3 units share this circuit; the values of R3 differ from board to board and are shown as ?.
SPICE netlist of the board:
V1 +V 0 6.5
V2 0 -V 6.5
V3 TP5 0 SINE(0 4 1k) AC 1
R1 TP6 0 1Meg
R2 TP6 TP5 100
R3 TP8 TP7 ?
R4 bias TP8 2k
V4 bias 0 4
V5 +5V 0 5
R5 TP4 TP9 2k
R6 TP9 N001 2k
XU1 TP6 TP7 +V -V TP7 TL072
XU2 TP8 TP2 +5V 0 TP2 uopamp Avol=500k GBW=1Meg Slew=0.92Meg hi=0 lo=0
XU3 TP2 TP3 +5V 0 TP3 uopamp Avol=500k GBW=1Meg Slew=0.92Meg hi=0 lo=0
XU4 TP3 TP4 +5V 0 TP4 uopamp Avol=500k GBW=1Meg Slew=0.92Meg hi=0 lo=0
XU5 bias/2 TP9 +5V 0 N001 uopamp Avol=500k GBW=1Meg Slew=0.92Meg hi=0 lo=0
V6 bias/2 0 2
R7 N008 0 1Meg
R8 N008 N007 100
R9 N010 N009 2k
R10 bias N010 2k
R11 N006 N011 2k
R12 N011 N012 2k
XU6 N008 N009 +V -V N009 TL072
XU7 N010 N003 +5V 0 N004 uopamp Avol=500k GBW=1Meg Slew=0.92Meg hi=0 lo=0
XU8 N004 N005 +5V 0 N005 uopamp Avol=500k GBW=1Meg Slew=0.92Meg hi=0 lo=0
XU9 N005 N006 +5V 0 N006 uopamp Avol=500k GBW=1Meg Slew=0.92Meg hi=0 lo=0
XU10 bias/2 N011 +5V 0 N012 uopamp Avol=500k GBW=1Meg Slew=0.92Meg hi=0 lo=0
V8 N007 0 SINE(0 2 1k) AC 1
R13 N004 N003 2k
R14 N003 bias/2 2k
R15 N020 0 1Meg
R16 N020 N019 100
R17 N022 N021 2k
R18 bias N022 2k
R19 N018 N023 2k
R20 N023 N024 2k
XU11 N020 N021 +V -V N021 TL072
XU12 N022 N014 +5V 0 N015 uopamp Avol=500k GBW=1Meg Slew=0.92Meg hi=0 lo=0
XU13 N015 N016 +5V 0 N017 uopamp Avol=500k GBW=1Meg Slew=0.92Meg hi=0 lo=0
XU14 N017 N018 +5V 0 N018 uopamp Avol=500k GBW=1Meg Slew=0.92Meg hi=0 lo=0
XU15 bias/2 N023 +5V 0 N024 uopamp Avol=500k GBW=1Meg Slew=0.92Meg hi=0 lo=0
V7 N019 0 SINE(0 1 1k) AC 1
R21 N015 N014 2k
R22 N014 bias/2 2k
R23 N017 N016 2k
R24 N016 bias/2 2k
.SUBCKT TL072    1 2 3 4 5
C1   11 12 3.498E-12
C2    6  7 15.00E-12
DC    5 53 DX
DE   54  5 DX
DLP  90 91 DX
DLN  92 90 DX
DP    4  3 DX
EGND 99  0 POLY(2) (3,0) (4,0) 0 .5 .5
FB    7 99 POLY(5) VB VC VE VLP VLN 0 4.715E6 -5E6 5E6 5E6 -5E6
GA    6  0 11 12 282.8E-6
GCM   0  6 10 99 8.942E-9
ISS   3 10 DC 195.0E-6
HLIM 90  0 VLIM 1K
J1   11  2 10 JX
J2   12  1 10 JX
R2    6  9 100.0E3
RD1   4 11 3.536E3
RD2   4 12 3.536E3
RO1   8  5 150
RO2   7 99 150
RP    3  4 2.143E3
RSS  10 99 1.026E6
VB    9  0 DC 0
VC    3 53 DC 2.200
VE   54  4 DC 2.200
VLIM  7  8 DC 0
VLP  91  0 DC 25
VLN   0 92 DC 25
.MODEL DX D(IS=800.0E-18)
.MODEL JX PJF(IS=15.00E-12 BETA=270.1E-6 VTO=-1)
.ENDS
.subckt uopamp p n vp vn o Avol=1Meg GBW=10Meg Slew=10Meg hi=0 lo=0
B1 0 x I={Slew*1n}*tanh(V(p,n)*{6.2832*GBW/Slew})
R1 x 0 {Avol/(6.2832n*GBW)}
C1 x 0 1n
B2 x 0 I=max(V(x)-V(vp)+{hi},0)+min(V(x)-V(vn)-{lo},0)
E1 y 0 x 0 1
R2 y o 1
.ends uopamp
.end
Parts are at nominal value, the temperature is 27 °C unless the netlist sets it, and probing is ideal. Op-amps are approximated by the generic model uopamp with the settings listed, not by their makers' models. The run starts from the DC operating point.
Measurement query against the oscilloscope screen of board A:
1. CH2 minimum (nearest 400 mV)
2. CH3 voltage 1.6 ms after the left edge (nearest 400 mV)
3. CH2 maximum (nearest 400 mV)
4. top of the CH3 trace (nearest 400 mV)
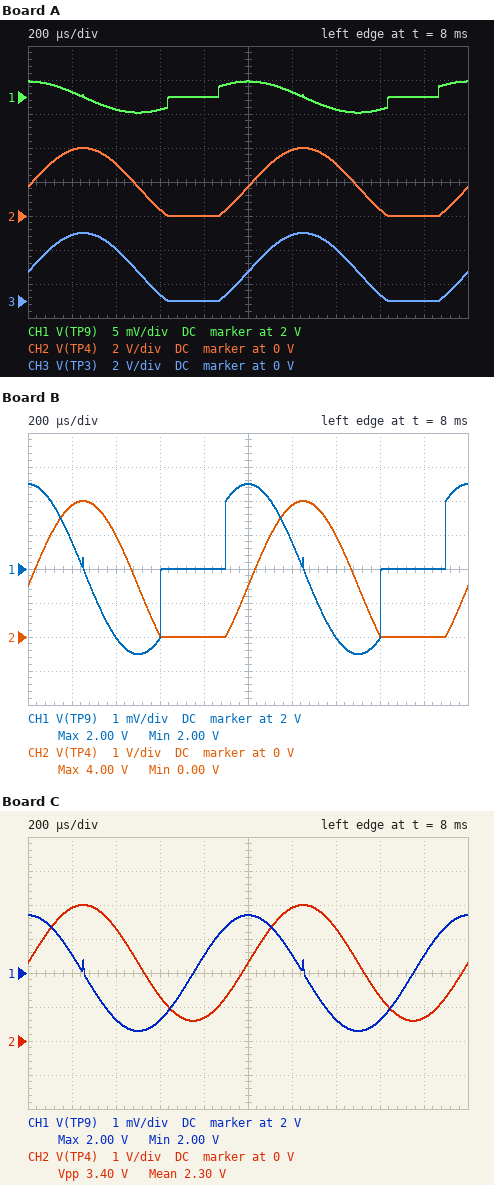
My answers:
0 V
400 mV
4.0 V
4.0 V
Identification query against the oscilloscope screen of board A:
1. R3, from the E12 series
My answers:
1.5 kΩ
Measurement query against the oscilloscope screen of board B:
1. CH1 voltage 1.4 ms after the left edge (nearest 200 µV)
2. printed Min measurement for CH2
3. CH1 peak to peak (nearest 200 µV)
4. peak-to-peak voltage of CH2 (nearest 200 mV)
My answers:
1.9980 V
0.00 V
5.0 mV
4.0 V
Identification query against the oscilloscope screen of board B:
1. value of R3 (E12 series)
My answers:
1.2 kΩ
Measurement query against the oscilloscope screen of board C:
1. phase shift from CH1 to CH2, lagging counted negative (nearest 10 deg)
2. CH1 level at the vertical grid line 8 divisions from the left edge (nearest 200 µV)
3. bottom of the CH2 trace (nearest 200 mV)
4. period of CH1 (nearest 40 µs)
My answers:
-90 deg
1.9986 V
600 mV
1.00 ms
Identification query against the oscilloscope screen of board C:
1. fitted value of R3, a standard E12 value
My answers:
2.7 kΩ
